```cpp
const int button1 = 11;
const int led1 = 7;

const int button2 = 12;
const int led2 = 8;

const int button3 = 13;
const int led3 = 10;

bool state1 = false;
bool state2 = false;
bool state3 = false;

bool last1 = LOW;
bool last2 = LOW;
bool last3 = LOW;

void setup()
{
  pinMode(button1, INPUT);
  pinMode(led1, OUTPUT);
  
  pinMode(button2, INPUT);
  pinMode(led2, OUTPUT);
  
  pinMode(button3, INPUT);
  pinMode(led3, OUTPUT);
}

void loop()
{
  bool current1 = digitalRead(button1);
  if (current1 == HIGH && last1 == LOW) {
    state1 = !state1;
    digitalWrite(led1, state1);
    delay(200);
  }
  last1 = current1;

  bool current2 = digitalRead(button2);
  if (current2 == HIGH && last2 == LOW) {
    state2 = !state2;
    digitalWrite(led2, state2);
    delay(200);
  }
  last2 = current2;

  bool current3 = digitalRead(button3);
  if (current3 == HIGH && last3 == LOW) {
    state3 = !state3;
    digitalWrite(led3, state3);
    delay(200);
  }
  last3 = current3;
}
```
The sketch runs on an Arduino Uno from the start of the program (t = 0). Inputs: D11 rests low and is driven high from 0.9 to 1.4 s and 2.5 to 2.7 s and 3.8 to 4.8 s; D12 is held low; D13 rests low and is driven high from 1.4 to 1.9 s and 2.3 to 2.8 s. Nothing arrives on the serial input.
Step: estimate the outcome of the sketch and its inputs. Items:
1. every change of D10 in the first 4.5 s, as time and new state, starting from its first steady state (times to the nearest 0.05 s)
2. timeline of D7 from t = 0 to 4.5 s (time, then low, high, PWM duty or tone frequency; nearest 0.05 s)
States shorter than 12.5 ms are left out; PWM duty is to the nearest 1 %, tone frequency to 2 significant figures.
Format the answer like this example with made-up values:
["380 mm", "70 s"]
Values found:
["0 s low; 1.4 s high; 2.3 s low", "0 s low; 0.9 s high; 2.5 s low; 3.8 s high"]
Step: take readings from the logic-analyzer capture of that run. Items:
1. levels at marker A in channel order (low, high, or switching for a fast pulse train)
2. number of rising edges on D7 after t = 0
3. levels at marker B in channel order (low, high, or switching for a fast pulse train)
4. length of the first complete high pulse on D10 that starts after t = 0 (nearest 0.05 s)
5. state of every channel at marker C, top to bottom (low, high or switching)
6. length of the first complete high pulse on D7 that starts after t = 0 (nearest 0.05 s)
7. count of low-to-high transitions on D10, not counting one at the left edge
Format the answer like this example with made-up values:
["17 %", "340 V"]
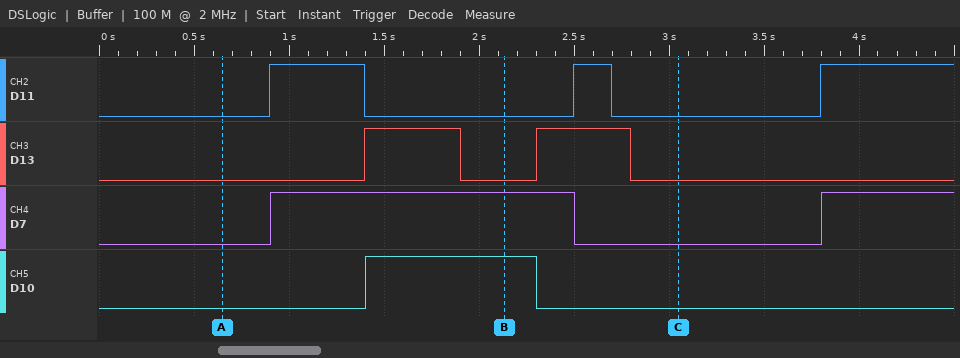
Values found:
["D11 low, D13 low, D7 low, D10 low", "2", "D11 low, D13 low, D7 high, D10 high", "0.90 s", "D11 low, D13 low, D7 low, D10 low", "1.60 s", "1"]
